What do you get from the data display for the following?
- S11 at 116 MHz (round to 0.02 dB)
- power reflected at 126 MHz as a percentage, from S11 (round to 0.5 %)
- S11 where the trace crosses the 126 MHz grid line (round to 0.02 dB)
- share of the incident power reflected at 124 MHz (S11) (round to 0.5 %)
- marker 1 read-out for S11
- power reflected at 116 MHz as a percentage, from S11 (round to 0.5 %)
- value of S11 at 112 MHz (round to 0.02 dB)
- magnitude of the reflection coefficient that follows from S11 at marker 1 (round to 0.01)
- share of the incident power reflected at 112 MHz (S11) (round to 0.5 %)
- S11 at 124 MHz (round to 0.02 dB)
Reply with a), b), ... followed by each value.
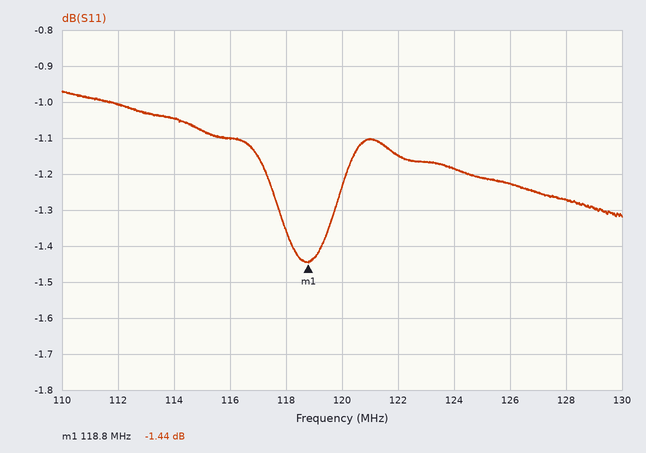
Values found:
a) -1.10 dB
b) 75.5 %
c) -1.22 dB
d) 76.0 %
e) -1.44 dB
f) 77.5 %
g) -1.00 dB
h) 0.85
i) 79.5 %
j) -1.18 dB
